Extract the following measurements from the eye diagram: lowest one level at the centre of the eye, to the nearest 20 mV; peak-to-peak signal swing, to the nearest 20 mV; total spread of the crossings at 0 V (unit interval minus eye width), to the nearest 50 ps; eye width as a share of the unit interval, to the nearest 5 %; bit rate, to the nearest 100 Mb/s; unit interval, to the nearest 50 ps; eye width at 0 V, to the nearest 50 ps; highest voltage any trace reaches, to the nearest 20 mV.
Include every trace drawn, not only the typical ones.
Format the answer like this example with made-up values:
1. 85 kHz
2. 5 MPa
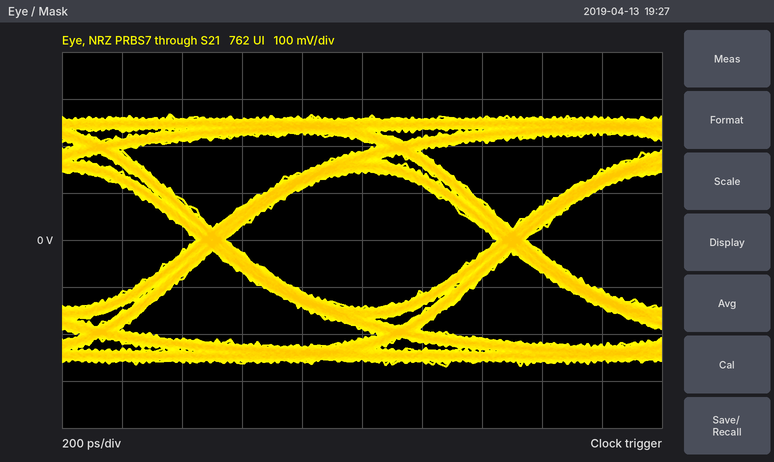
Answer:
1. 140 mV
2. 540 mV
3. 100 ps
4. 90 %
5. 1.0 Gb/s
6. 1.00 ns
7. 900 ps
8. 260 mV
